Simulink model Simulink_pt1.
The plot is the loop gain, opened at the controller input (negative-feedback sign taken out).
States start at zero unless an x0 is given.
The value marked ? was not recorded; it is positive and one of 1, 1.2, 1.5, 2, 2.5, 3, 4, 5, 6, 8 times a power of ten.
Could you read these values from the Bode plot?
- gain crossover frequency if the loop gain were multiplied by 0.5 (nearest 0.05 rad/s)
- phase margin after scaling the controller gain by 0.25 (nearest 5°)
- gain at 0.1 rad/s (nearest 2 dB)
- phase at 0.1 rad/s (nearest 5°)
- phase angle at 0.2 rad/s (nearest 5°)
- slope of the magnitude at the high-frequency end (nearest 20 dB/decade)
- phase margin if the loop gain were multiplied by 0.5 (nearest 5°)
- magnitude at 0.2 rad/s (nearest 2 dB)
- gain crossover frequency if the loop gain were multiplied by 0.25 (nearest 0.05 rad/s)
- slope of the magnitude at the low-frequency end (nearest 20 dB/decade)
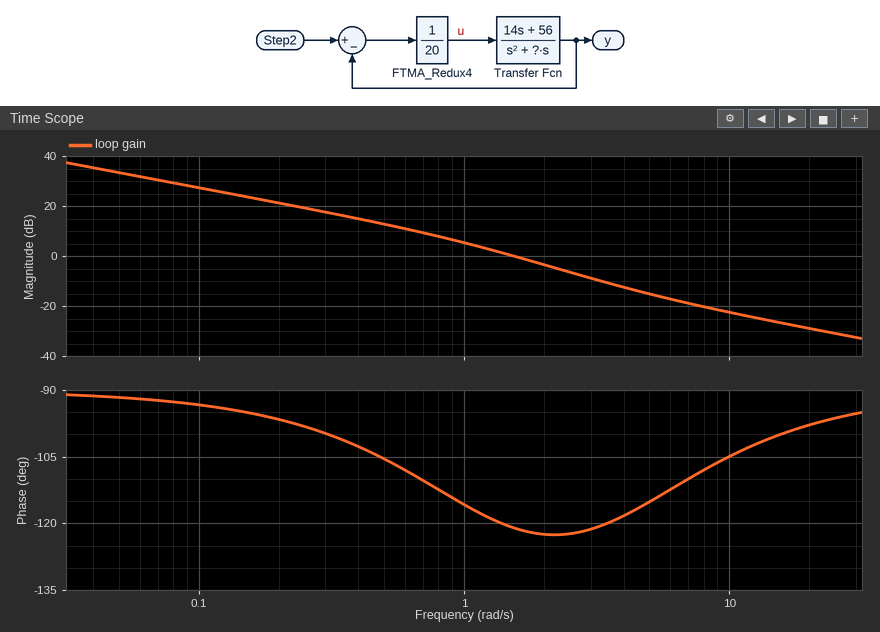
0.95 rad/s
75°
28 dB
-95°
-95°
-20 dB/decade
65°
22 dB
0.55 rad/s
-20 dB/decade
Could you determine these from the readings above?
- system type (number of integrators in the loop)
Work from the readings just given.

1
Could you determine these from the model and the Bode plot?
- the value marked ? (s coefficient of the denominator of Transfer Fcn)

1.2
